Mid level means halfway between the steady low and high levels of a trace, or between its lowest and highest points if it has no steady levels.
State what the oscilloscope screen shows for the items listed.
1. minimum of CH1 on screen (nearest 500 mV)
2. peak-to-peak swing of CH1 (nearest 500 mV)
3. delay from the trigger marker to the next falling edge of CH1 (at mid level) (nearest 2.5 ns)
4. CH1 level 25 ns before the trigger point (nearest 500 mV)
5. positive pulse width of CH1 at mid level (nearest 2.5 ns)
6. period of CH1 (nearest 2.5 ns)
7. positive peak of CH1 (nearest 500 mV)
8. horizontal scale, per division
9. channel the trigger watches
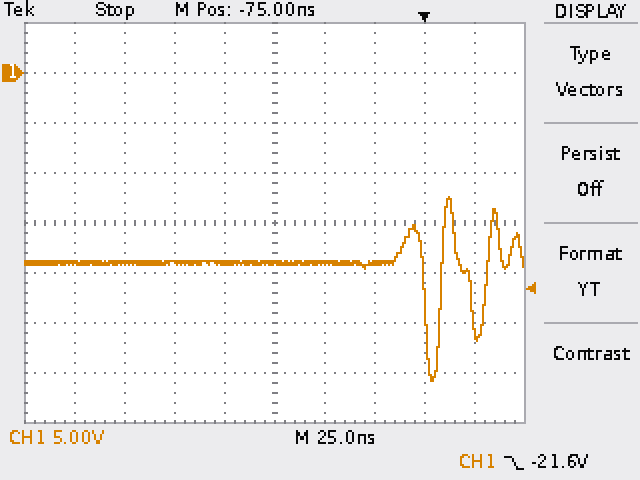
-31.0 V
18.5 V
22.5 ns
-19.0 V
15.0 ns
22.5 ns
-12.5 V
25 ns
CH1
